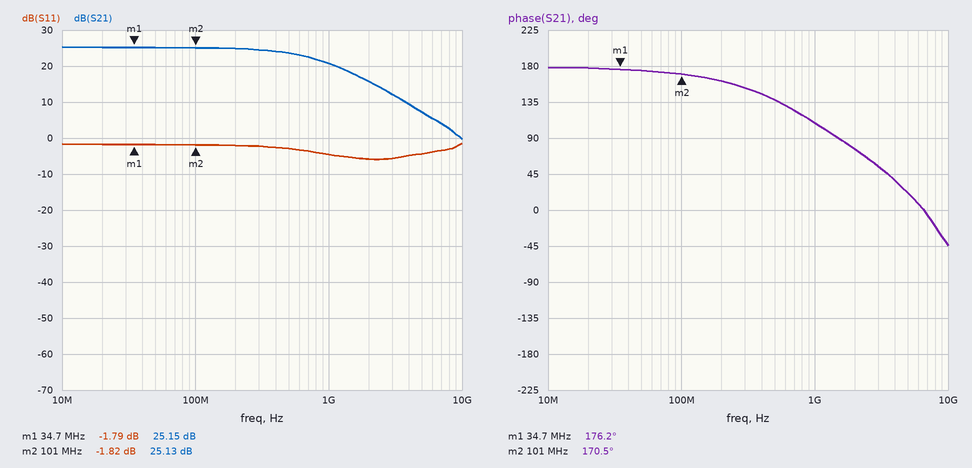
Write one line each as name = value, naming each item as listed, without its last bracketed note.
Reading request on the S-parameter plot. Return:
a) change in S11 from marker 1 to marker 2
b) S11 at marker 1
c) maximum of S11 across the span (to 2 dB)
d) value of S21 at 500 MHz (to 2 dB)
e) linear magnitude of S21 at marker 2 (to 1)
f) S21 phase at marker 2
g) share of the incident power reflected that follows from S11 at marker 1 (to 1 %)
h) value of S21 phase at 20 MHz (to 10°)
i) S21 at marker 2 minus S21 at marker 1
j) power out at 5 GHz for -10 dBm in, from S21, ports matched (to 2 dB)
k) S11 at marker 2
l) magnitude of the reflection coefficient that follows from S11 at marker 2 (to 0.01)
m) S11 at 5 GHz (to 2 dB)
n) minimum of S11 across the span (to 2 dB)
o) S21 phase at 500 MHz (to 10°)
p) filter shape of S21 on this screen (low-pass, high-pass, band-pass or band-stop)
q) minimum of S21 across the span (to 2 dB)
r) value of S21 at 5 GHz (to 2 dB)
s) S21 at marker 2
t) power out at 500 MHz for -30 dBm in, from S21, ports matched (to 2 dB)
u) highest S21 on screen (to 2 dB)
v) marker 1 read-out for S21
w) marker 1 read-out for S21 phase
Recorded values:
change in S11 from marker 1 to marker 2 = -0.03 dB
S11 at marker 1 = -1.79 dB
maximum of S11 across the span = -2 dB
value of S21 at 500 MHz = 24 dB
linear magnitude of S21 at marker 2 = 18
S21 phase at marker 2 = 170.5°
share of the incident power reflected that follows from S11 at marker 1 = 66 %
value of S21 phase at 20 MHz = 180°
S21 at marker 2 minus S21 at marker 1 = -0.02 dB
power out at 5 GHz for -10 dBm in, from S21, ports matched = -2 dBm
S11 at marker 2 = -1.82 dB
magnitude of the reflection coefficient that follows from S11 at marker 2 = 0.81
S11 at 5 GHz = -4 dB
minimum of S11 across the span = -6 dB
S21 phase at 500 MHz = 140°
filter shape of S21 on this screen = low-pass
minimum of S21 across the span = 0 dB
value of S21 at 5 GHz = 8 dB
S21 at marker 2 = 25.13 dB
power out at 500 MHz for -30 dBm in, from S21, ports matched = -6 dBm
highest S21 on screen = 26 dB
marker 1 read-out for S21 = 25.15 dB
marker 1 read-out for S21 phase = 176.2°
